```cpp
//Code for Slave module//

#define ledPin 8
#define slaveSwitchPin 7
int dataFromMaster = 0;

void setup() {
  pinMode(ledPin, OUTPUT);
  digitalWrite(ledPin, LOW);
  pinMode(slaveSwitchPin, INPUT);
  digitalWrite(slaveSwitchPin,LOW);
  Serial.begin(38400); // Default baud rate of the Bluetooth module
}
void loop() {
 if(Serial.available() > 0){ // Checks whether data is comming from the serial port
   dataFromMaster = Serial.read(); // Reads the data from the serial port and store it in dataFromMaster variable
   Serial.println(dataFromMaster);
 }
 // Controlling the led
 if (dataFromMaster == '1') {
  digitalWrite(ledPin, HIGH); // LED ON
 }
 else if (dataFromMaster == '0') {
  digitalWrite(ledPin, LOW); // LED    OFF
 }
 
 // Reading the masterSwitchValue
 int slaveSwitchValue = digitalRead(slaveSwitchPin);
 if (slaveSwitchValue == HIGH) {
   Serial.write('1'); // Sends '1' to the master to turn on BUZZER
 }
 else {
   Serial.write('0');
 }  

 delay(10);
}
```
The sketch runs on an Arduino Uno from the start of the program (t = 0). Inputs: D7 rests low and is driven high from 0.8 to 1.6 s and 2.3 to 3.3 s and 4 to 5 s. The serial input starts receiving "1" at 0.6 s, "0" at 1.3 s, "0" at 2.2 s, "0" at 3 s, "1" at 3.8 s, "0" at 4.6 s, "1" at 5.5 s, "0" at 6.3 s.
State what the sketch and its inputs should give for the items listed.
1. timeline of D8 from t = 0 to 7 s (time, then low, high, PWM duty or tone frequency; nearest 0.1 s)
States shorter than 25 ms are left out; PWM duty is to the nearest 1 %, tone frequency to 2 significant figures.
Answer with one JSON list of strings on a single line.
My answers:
["0 s low; 0.6 s high; 1.3 s low; 3.8 s high; 4.6 s low; 5.5 s high; 6.3 s low"]
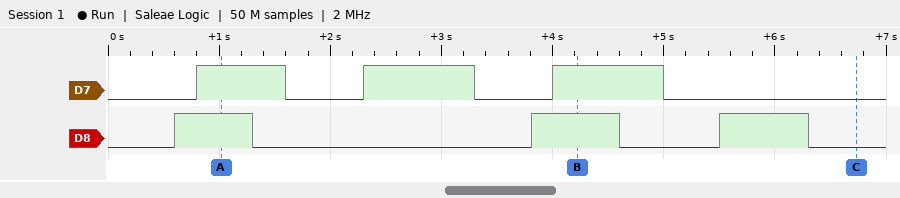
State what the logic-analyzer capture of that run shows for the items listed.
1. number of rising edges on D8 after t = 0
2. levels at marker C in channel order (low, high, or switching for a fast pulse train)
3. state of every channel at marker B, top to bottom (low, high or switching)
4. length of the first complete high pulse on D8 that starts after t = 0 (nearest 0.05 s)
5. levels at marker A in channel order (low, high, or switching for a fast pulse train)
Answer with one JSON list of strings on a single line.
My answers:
["3", "D7 low, D8 low", "D7 high, D8 high", "0.70 s", "D7 high, D8 high"]
